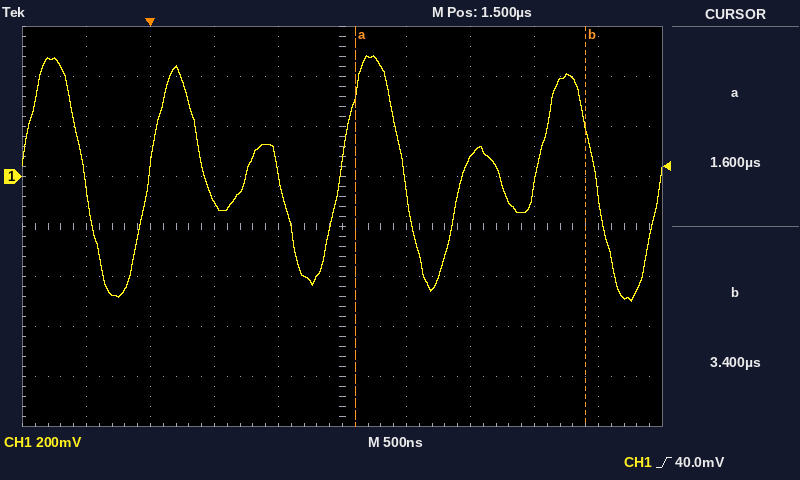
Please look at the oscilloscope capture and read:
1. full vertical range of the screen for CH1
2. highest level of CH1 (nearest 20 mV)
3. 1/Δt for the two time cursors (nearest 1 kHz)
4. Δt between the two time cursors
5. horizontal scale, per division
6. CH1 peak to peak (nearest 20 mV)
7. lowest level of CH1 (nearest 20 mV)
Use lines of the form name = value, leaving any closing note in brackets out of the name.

full vertical range of the screen for CH1 = 1.6 V
highest level of CH1 = 480 mV
1/Δt for the two time cursors = 556 kHz
Δt between the two time cursors = 1.80 µs
horizontal scale, per division = 500 ns
CH1 peak to peak = 980 mV
lowest level of CH1 = -500 mV
